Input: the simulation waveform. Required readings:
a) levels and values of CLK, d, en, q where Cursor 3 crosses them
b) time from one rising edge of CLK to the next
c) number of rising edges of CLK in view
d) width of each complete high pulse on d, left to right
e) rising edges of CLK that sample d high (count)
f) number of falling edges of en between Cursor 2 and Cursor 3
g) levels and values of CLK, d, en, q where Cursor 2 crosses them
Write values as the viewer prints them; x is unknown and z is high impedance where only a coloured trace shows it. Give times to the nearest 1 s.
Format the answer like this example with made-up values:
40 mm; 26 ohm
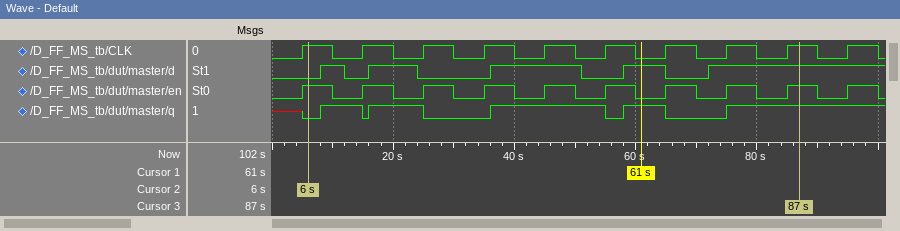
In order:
CLK=1, d=1, en=1, q=1; 10 s; 10; 4 s, 8 s, 15 s, 7 s; 5; 8; CLK=1, d=0, en=1, q=0
